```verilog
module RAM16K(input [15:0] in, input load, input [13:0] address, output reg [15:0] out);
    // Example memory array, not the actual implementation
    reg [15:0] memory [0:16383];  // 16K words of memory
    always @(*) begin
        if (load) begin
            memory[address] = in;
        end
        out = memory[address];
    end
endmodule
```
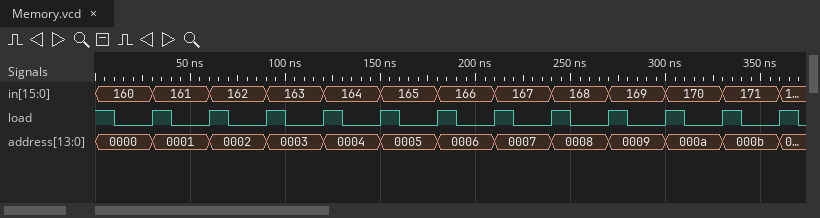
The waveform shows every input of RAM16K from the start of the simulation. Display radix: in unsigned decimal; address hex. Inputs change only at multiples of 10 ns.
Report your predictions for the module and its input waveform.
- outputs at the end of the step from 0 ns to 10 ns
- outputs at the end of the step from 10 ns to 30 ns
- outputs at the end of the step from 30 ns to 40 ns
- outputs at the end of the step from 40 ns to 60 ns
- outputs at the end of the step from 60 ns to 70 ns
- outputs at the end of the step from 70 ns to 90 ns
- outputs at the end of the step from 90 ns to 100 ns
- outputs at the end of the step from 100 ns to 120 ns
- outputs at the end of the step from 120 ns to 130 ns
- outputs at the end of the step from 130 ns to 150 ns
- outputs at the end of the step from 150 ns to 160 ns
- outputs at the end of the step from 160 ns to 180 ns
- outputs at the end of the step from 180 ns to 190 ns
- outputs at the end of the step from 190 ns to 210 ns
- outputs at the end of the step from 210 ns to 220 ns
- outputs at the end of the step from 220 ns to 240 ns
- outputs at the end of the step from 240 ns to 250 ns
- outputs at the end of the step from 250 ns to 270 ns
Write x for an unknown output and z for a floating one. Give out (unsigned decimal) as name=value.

out=160
out=160
out=161
out=161
out=162
out=162
out=163
out=163
out=164
out=164
out=165
out=165
out=166
out=166
out=167
out=167
out=168
out=168
